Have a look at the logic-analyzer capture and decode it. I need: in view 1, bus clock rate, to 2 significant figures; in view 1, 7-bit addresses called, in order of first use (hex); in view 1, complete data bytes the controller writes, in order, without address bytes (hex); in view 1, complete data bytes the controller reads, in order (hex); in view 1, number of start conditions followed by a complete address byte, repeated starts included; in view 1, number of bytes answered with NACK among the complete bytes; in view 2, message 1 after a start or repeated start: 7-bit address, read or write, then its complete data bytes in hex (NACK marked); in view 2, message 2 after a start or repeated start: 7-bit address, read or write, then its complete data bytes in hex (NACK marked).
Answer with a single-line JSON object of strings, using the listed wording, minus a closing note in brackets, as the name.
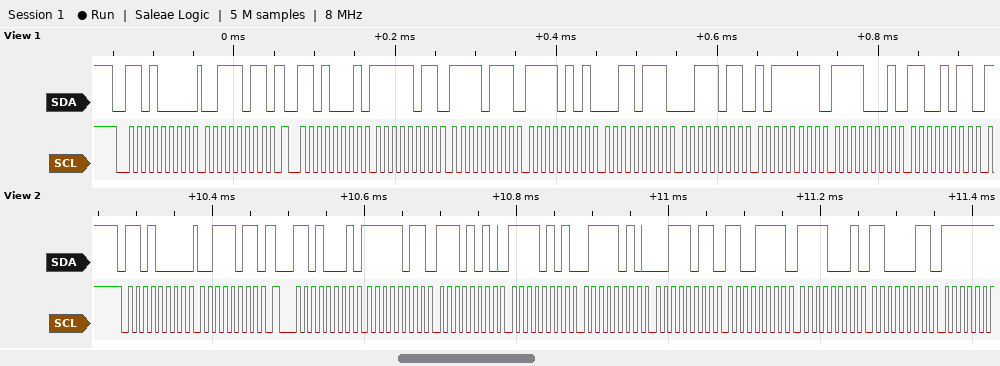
{"in view 1, bus clock rate, to 2 significant figures": "100 kHz", "in view 1, 7-bit addresses called, in order of first use": "0x68", "in view 1, complete data bytes the controller writes, in order, without address bytes": "3B", "in view 1, complete data bytes the controller reads, in order": "FB F7 F5 37 3B BF F1 CB", "in view 1, number of start conditions followed by a complete address byte, repeated starts included": "2", "in view 1, number of bytes answered with NACK among the complete bytes": "0", "in view 2, message 1 after a start or repeated start: 7-bit address, read or write, then its complete data bytes in hex": "0x68 write: 3B", "in view 2, message 2 after a start or repeated start: 7-bit address, read or write, then its complete data bytes in hex": "0x68 read: FB EA F5 7A 3B CF F1 C3"}
